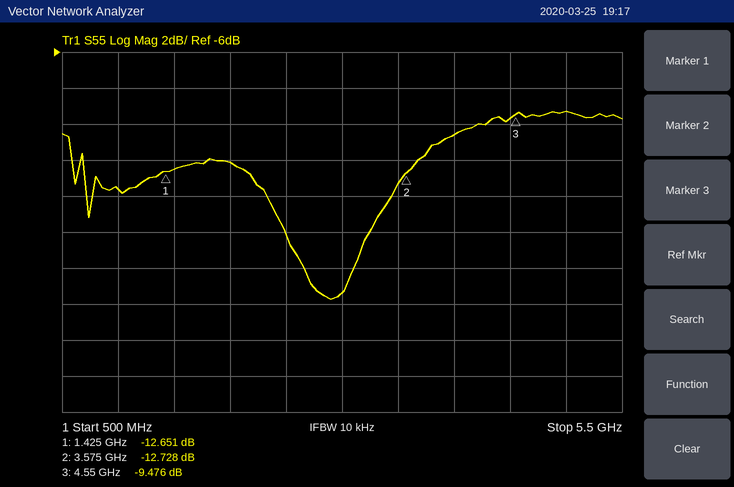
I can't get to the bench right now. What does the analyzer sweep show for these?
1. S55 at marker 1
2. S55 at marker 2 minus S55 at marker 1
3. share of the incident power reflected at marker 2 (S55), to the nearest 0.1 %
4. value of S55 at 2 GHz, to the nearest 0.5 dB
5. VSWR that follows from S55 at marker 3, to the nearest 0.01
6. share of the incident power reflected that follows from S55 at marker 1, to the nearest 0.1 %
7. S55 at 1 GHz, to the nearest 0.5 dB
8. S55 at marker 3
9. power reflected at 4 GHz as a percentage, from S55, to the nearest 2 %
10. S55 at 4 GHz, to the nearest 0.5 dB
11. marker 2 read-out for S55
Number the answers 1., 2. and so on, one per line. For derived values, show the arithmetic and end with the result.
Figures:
1. -12.651 dB
2. -12.728 − (-12.651) = -0.077 dB
3. 10^(-12.728/10) ≈ 5.3 %
4. -12.0 dB
5. (1 + 0.3359)/(1 − 0.3359) ≈ 2.01
6. 10^(-12.651/10) ≈ 5.4 %
7. -13.5 dB
8. -9.476 dB
9. 10^(-10.5/10) ≈ 8.91 %, so 8 % to the nearest 2 %
10. -10.5 dB
11. -12.728 dB
